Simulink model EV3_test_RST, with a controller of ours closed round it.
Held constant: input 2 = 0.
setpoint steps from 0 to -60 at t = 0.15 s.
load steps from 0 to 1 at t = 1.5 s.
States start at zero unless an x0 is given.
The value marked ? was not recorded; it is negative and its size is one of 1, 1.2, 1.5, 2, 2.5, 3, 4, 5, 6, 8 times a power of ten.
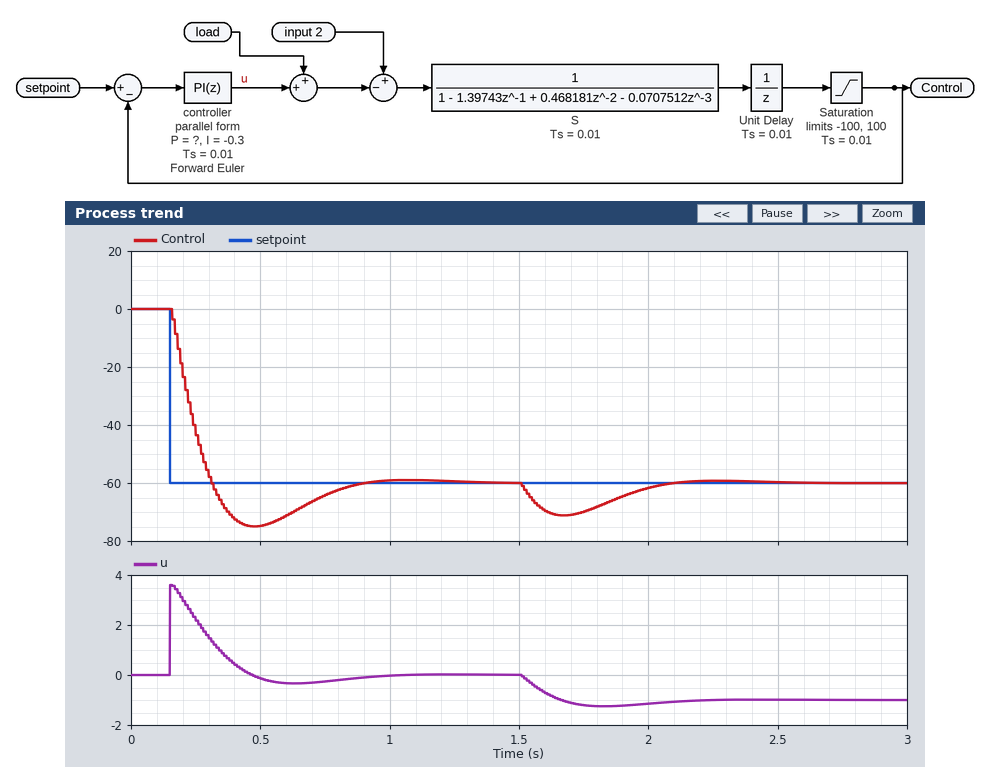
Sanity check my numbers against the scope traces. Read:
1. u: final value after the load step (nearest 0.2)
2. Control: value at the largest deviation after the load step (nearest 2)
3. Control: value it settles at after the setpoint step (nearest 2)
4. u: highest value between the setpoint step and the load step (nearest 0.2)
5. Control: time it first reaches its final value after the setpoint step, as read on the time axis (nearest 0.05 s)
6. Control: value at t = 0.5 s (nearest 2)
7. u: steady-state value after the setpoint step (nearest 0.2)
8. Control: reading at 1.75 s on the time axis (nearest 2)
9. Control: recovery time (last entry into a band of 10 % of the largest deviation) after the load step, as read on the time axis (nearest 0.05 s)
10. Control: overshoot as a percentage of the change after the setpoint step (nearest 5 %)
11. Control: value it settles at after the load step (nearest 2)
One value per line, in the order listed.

-1.0
-72
-60
3.6
0.30 s
-74
0.0
-70
2.05 s
25 %
-60
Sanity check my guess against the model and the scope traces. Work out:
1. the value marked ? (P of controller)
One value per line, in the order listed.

-0.06
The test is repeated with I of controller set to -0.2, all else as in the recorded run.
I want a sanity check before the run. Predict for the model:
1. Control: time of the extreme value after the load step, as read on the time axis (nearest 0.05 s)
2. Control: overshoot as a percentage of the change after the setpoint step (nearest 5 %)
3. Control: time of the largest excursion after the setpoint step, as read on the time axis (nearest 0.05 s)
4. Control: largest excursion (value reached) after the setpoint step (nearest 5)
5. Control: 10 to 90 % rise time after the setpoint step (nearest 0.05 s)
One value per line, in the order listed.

1.70 s
20 %
0.50 s
-70
0.15 s
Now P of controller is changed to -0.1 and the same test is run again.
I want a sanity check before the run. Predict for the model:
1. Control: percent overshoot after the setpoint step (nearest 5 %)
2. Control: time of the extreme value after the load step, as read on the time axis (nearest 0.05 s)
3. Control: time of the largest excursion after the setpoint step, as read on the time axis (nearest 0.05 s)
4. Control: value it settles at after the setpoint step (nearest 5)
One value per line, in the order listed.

15 %
1.65 s
0.40 s
-60
